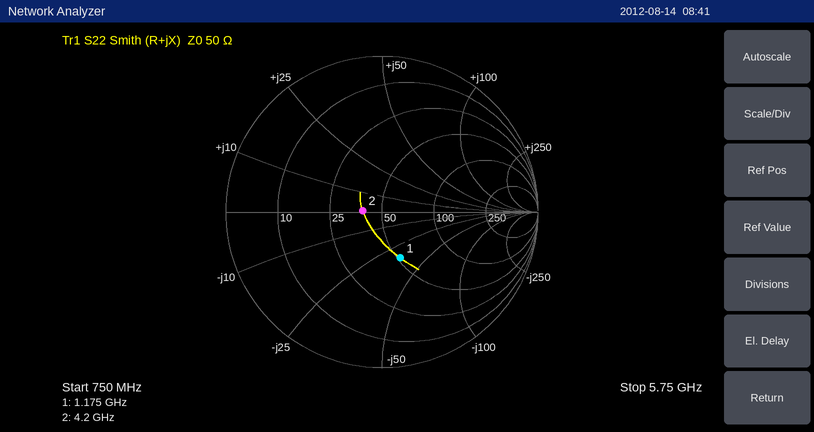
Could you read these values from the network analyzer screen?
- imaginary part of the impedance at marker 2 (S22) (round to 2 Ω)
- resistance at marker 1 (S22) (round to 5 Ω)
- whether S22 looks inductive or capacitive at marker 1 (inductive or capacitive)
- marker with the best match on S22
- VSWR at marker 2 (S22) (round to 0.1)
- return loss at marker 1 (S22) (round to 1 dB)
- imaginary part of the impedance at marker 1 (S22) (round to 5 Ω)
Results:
0 Ω
50 Ω
capacitive
marker 2
1.3
10 dB
-35 Ω
